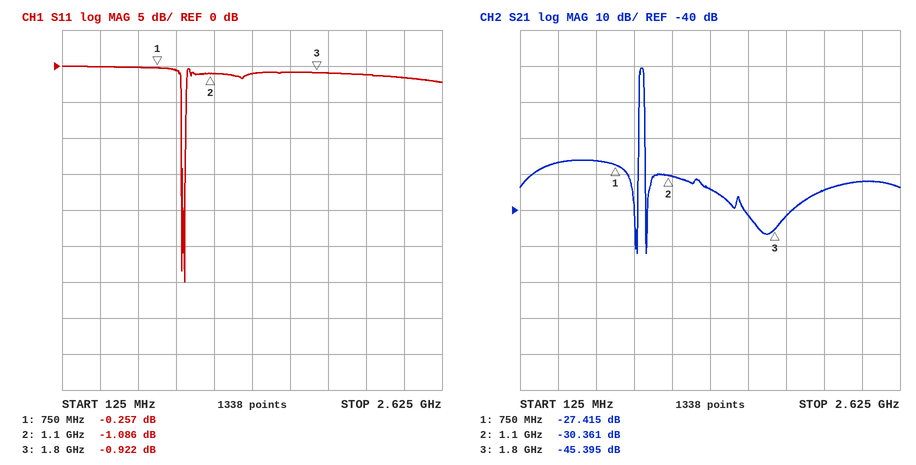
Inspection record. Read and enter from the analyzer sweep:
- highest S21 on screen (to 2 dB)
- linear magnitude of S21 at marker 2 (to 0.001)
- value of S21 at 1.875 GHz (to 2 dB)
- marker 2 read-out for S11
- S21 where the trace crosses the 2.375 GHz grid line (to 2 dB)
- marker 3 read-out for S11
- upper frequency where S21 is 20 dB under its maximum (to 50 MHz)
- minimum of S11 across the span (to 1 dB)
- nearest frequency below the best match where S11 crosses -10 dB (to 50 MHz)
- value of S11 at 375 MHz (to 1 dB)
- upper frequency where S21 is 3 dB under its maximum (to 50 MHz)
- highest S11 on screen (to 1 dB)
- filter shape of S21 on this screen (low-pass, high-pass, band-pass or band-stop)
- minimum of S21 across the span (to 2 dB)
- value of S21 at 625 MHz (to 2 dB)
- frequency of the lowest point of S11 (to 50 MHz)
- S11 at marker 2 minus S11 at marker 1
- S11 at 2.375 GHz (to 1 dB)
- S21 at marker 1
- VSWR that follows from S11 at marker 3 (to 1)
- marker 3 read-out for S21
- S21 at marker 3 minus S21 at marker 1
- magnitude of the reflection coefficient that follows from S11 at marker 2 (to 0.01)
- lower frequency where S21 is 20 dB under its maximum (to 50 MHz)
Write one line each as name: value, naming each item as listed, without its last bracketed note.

highest S21 on screen: 0 dB
linear magnitude of S21 at marker 2: 0.030
value of S21 at 1.875 GHz: -42 dB
marker 2 read-out for S11: -1.086 dB
S21 where the trace crosses the 2.375 GHz grid line: -32 dB
marker 3 read-out for S11: -0.922 dB
upper frequency where S21 is 20 dB under its maximum: 950 MHz
minimum of S11 across the span: -30 dB
nearest frequency below the best match where S11 crosses -10 dB: 900 MHz
value of S11 at 375 MHz: 0 dB
upper frequency where S21 is 3 dB under its maximum: 950 MHz
highest S11 on screen: 0 dB
filter shape of S21 on this screen: band-pass
minimum of S21 across the span: -52 dB
value of S21 at 625 MHz: -26 dB
frequency of the lowest point of S11: 950 MHz
S11 at marker 2 minus S11 at marker 1: -0.829 dB
S11 at 2.375 GHz: -2 dB
S21 at marker 1: -27.415 dB
VSWR that follows from S11 at marker 3: 19
marker 3 read-out for S21: -45.395 dB
S21 at marker 3 minus S21 at marker 1: -17.980 dB
magnitude of the reflection coefficient that follows from S11 at marker 2: 0.88
lower frequency where S21 is 20 dB under its maximum: 900 MHz
